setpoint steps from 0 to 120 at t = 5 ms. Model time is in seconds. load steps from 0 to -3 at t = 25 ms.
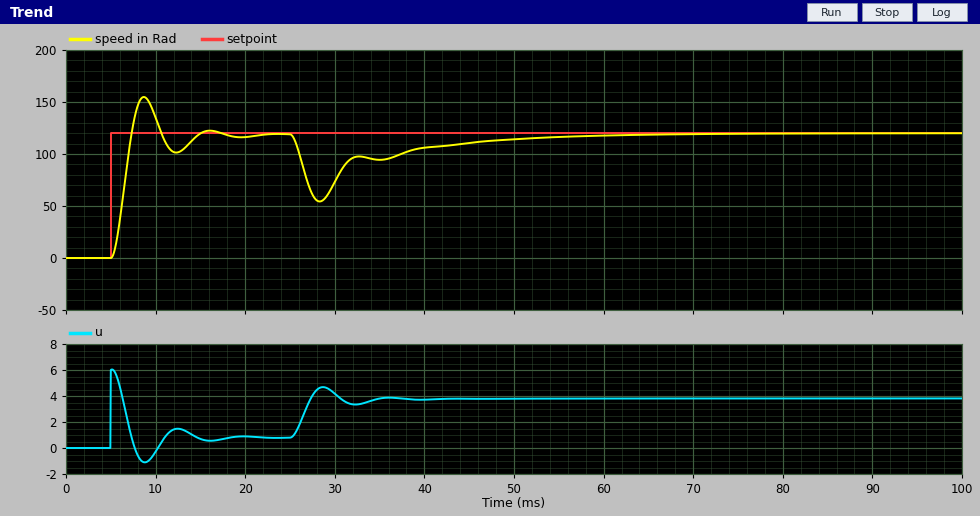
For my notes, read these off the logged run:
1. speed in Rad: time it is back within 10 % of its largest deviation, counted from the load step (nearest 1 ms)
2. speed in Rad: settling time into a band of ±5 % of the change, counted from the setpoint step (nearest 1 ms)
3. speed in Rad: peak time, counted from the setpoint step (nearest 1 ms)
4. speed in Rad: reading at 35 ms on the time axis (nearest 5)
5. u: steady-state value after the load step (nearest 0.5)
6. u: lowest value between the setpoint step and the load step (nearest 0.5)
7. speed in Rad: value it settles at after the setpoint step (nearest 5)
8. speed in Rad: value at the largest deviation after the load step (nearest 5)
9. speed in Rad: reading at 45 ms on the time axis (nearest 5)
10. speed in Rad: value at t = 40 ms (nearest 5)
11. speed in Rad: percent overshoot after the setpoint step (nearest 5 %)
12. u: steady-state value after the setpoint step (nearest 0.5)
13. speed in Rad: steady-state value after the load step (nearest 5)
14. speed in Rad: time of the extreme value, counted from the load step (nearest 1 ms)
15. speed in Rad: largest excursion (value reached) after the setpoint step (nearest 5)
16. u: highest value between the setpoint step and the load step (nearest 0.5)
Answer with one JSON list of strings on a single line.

["24 ms", "9 ms", "4 ms", "95", "4.0", "-1.0", "120", "55", "110", "105", "30 %", "1.0", "120", "3 ms", "155", "6.0"]
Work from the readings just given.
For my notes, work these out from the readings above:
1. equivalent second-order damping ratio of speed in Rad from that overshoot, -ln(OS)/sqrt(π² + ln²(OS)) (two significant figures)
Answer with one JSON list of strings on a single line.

["0.36"]
